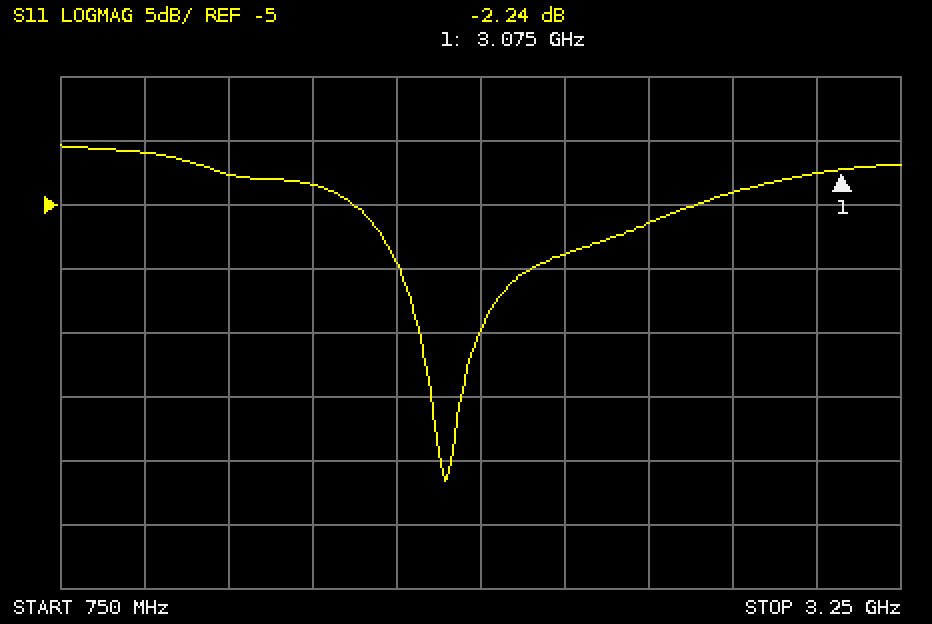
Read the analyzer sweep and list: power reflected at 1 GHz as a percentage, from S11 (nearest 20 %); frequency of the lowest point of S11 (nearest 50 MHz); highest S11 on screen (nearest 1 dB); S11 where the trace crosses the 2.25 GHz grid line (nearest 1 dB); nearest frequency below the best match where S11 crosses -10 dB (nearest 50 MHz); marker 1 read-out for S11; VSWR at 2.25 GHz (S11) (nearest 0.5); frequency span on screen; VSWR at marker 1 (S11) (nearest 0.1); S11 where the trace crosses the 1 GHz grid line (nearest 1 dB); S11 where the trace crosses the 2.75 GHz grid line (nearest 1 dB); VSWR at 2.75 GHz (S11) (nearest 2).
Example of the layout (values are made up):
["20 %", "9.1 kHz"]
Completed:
["80 %", "1.90 GHz", "0 dB", "-9 dB", "1.75 GHz", "-2.24 dB", "2.0", "2.5 GHz", "7.8", "-1 dB", "-4 dB", "4"]
